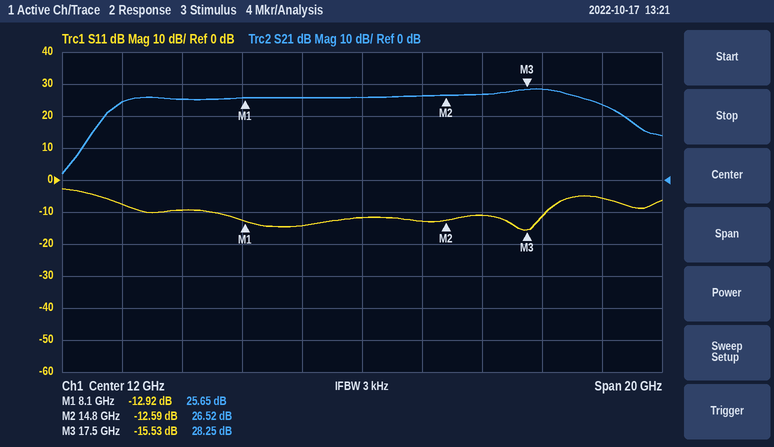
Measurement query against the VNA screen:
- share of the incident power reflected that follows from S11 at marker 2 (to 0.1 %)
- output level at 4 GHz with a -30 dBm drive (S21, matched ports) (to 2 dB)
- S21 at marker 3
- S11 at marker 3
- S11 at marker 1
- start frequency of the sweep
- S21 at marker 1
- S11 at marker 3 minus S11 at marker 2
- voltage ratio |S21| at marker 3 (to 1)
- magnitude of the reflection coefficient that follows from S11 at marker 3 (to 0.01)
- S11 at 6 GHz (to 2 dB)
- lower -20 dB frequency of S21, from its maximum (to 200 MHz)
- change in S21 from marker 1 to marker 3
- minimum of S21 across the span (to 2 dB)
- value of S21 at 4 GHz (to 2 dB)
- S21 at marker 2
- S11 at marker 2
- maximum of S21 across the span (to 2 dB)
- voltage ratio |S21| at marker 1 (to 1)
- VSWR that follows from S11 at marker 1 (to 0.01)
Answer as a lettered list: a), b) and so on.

a) 5.5 %
b) -6 dBm
c) 28.25 dB
d) -15.53 dB
e) -12.92 dB
f) 2 GHz
g) 25.65 dB
h) -2.94 dB
i) 26
j) 0.17
k) -10 dB
l) 2.6 GHz
m) 2.60 dB
n) 2 dB
o) 24 dB
p) 26.52 dB
q) -12.59 dB
r) 28 dB
s) 19
t) 1.58
